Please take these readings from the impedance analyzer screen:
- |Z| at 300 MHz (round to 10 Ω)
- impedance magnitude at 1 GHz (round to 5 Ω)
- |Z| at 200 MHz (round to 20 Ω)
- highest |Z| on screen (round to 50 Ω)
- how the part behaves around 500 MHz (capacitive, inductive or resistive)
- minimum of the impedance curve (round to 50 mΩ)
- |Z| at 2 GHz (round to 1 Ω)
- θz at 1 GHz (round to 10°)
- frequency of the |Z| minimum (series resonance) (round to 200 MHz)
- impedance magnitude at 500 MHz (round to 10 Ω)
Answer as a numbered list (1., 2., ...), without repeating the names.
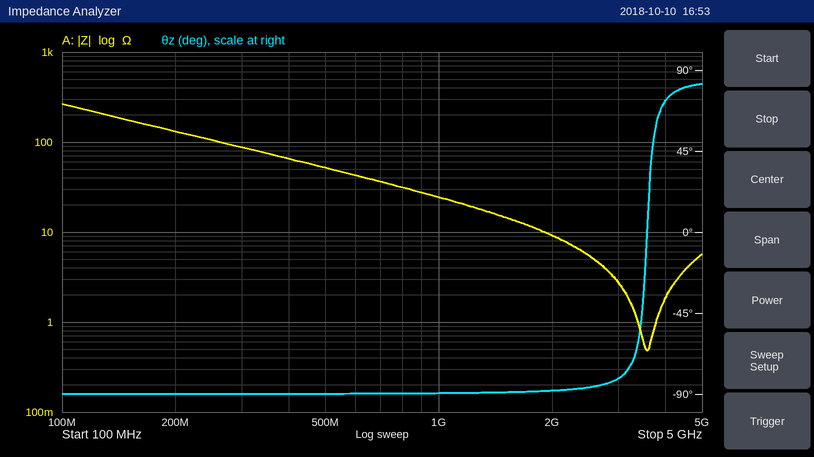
1. 90 Ω
2. 25 Ω
3. 140 Ω
4. 250 Ω
5. capacitive
6. 500 mΩ
7. 9 Ω
8. -90°
9. 3.6 GHz
10. 50 Ω
